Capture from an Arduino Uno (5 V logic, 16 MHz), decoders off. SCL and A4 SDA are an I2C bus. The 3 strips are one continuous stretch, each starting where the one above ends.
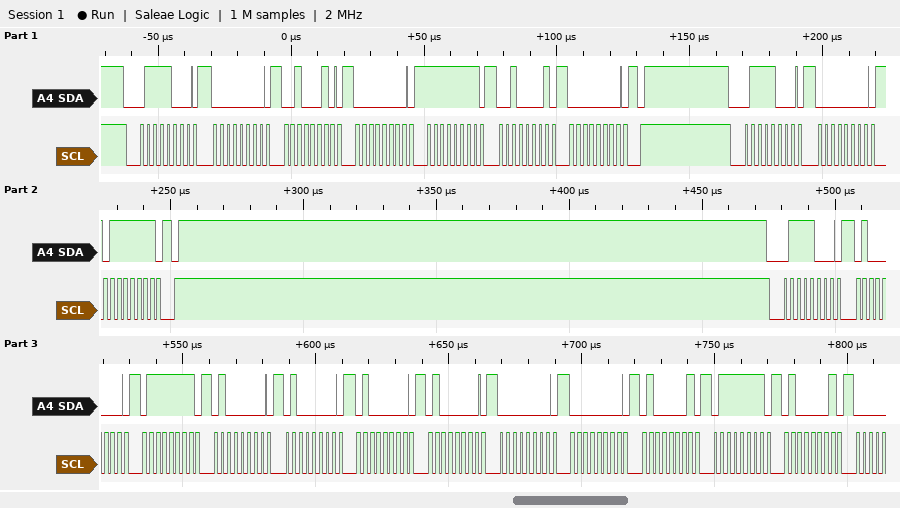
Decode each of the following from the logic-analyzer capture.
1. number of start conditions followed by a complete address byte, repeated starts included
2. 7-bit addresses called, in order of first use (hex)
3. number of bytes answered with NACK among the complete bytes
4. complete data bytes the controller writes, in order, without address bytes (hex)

3
0x3C
0
00 22 00 FF 21 00 00 7F 40 7F 40 40 40 40 00 00 41 7F 41
